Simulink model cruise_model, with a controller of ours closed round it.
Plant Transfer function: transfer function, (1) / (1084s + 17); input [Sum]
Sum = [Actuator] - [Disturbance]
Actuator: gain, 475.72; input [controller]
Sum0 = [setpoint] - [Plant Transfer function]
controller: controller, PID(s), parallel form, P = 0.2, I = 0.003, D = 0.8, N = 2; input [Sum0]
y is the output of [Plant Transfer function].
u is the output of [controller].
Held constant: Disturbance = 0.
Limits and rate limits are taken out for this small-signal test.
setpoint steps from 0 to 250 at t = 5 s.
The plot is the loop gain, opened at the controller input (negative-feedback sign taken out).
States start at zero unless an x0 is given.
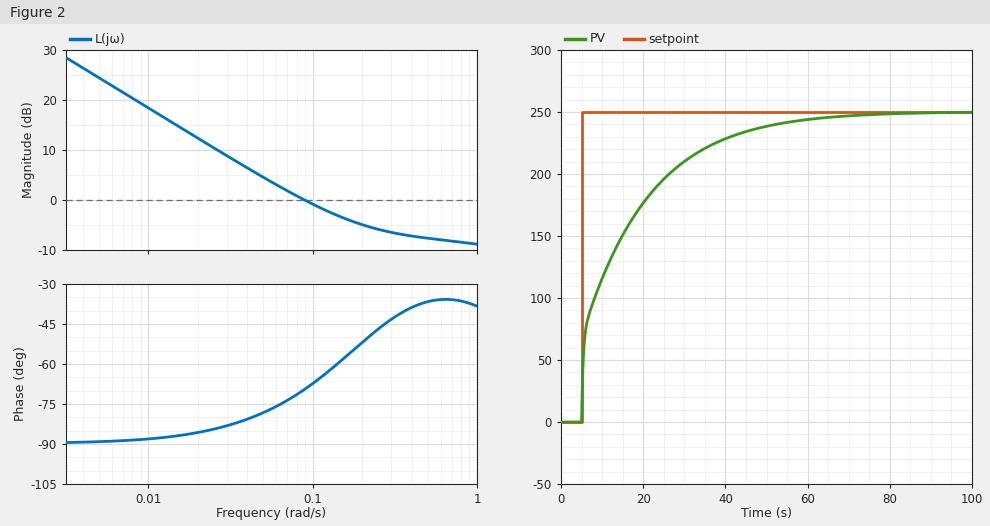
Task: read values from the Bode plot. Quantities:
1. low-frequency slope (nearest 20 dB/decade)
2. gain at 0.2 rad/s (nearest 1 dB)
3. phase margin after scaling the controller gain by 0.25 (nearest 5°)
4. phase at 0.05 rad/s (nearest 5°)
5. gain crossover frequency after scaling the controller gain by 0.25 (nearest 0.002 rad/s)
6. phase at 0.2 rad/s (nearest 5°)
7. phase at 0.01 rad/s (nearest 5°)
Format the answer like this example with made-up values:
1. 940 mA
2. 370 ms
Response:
1. -20 dB/decade
2. -5 dB
3. 95°
4. -80°
5. 0.020 rad/s
6. -50°
7. -90°
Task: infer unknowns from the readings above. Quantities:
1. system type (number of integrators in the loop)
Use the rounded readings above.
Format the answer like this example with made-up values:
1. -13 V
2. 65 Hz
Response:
1. 1
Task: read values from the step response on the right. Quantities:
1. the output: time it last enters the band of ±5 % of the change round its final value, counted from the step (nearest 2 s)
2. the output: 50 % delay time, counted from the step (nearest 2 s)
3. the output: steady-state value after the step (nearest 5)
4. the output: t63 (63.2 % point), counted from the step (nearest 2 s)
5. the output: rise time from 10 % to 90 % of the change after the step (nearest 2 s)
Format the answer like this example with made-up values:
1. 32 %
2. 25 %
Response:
1. 44 s
2. 6 s
3. 250
4. 12 s
5. 32 s
